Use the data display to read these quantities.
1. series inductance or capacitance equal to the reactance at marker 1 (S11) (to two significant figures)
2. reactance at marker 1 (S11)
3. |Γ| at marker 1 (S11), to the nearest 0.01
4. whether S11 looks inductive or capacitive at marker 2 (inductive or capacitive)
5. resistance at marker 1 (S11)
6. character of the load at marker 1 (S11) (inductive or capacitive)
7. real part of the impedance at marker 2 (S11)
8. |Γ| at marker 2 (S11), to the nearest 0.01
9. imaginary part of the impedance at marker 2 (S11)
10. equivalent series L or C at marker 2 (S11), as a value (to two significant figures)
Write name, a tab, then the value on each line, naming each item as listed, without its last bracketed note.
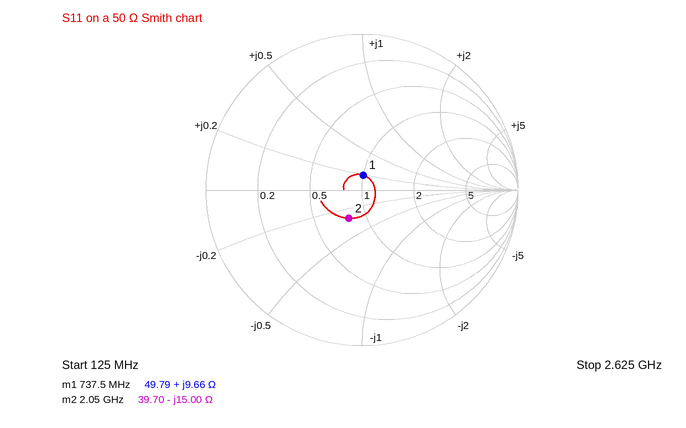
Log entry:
series inductance or capacitance equal to the reactance at marker 1 (S11)	2.1 nH
reactance at marker 1	+9.66 Ω
|Γ| at marker 1 (S11), to the nearest 0.01	0.10
whether S11 looks inductive or capacitive at marker 2	capacitive
resistance at marker 1	49.79 Ω
character of the load at marker 1 (S11)	inductive
real part of the impedance at marker 2	39.70 Ω
|Γ| at marker 2 (S11), to the nearest 0.01	0.20
imaginary part of the impedance at marker 2	-15.00 Ω
equivalent series L or C at marker 2 (S11), as a value	5.2 pF
